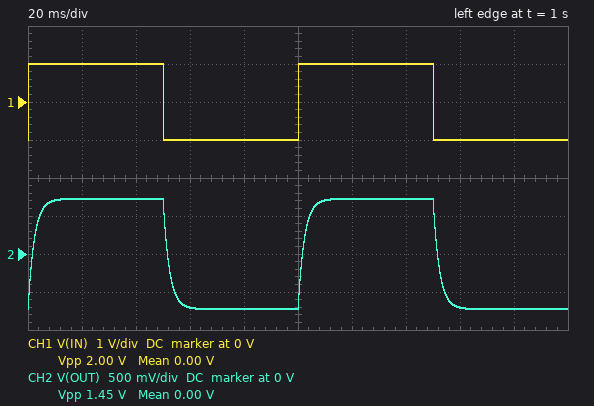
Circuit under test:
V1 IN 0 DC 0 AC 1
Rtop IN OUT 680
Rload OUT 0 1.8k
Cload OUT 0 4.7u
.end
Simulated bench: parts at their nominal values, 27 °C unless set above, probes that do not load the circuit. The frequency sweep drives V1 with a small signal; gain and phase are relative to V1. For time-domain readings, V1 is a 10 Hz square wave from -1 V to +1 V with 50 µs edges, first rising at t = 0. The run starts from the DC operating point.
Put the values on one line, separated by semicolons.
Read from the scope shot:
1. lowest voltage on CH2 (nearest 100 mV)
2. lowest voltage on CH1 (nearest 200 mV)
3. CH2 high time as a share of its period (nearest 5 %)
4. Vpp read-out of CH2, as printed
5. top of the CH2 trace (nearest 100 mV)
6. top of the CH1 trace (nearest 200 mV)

-700 mV; -1.0 V; 50 %; 1.45 V; 700 mV; 1.0 V
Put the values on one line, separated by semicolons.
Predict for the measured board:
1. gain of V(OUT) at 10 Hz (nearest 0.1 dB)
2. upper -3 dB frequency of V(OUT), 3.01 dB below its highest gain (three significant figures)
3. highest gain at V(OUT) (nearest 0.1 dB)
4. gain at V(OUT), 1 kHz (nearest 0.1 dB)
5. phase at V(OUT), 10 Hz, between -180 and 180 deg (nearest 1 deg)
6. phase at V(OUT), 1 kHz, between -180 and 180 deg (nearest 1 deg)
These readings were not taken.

-2.9 dB; 68.6 Hz; -2.8 dB; -26.1 dB; -8 deg; -86 deg
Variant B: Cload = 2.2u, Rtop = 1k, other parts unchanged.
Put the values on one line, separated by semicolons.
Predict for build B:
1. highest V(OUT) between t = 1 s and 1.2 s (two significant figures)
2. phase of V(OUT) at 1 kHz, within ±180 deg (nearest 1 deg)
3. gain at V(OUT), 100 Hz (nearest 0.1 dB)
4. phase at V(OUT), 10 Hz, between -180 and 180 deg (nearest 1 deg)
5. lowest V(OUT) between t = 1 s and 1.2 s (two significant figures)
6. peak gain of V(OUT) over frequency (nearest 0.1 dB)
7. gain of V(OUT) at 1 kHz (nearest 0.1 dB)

640 mV; -84 deg; -6.4 dB; -5 deg; -640 mV; -3.8 dB; -22.9 dB
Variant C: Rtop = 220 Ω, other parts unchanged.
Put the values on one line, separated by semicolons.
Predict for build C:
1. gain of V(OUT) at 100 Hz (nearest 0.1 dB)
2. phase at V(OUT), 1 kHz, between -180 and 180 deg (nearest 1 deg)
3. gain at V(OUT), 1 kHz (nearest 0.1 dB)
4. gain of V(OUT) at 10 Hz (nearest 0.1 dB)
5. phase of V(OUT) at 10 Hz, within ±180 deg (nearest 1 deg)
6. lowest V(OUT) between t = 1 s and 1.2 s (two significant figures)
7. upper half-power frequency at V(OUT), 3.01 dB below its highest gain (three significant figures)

-2.3 dB; -80 deg; -16.4 dB; -1.0 dB; -3 deg; -890 mV; 173 Hz
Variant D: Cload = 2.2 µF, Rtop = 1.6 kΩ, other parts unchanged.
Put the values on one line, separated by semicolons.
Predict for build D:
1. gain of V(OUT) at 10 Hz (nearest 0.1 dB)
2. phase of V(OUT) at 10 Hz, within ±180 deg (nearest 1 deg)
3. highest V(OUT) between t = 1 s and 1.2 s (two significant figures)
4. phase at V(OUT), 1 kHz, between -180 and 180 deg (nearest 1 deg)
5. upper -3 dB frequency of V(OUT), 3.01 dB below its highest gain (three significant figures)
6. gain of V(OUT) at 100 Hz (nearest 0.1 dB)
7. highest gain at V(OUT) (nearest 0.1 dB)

-5.6 dB; -7 deg; 530 mV; -85 deg; 85.4 Hz; -9.3 dB; -5.5 dB
